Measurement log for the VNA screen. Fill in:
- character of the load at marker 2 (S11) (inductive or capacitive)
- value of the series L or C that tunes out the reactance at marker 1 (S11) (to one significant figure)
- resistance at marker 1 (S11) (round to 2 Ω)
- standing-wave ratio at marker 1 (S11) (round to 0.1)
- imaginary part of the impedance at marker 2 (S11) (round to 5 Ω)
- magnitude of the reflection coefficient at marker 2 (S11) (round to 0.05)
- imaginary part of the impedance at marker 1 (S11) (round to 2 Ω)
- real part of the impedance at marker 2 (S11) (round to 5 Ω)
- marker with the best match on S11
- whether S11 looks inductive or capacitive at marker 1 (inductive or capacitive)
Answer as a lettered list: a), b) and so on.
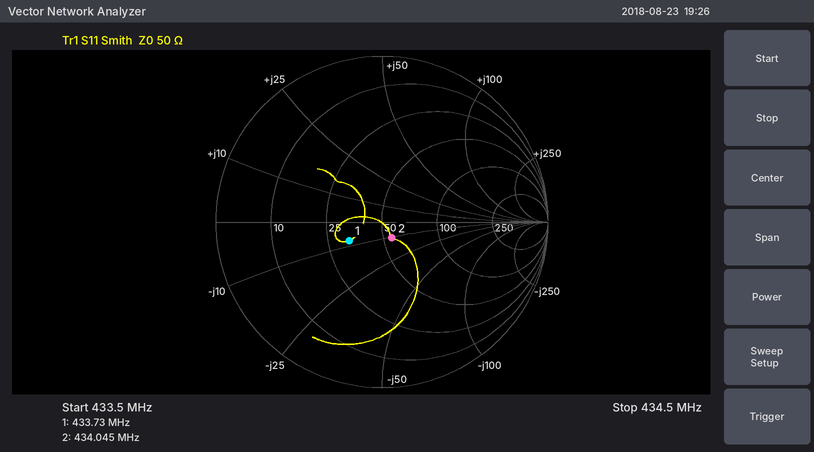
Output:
a) capacitive
b) 3 nH
c) 32 Ω
d) 1.6
e) -10 Ω
f) 0.10
g) -8 Ω
h) 55 Ω
i) marker 2
j) capacitive
